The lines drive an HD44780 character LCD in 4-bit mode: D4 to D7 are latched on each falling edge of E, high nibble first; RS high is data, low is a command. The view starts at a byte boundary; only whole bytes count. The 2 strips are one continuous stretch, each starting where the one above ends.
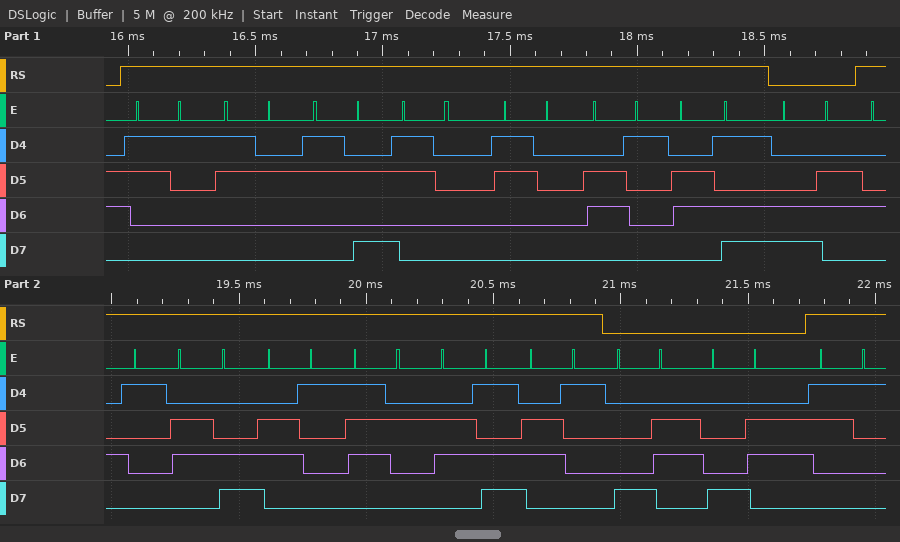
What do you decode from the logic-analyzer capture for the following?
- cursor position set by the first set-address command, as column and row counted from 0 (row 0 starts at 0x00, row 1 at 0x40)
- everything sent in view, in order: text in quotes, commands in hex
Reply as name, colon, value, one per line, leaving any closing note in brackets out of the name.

cursor position set by the first set-address command, as column and row counted from 0: column 6, row 1
everything sent in view, in order: text in quotes, commands in hex: "12:00am" 0xC6 "Alarma" 0x86 0x86 "1"
